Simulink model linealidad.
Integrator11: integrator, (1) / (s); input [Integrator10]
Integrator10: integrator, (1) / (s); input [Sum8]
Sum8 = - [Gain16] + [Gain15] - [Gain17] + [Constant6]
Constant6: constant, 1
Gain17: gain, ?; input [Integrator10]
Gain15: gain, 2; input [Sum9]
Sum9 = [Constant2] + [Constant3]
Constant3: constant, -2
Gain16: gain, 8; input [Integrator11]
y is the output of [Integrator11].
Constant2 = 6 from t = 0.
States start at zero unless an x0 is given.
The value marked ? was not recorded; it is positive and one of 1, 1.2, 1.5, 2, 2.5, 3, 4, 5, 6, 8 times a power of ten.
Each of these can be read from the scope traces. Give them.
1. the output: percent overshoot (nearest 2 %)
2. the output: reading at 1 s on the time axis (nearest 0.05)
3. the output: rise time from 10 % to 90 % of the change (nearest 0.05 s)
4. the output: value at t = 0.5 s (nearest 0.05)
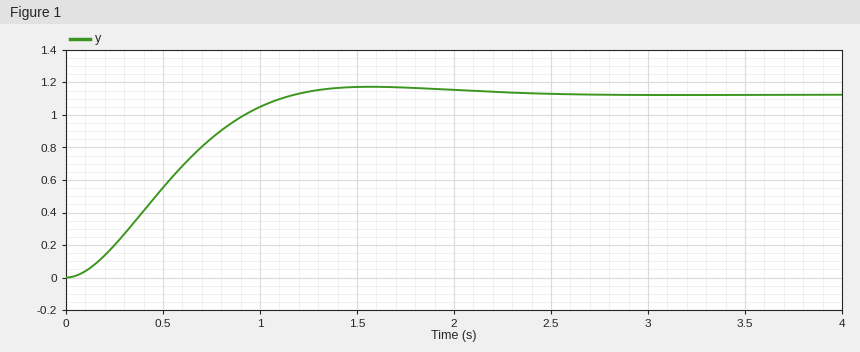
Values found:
4 %
1.05
0.75 s
0.55
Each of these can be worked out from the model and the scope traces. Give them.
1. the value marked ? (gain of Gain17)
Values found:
4
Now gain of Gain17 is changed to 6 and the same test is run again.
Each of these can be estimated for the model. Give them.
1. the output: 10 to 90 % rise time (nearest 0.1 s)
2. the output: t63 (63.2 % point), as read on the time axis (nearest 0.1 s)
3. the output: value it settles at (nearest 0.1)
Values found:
1.3 s
0.8 s
1.1
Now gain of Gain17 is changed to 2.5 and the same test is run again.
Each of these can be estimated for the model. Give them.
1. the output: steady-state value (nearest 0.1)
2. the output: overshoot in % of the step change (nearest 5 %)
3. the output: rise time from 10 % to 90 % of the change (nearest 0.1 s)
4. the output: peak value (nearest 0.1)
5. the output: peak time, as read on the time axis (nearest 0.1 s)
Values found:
1.1
20 %
0.5 s
1.4
1.2 s
